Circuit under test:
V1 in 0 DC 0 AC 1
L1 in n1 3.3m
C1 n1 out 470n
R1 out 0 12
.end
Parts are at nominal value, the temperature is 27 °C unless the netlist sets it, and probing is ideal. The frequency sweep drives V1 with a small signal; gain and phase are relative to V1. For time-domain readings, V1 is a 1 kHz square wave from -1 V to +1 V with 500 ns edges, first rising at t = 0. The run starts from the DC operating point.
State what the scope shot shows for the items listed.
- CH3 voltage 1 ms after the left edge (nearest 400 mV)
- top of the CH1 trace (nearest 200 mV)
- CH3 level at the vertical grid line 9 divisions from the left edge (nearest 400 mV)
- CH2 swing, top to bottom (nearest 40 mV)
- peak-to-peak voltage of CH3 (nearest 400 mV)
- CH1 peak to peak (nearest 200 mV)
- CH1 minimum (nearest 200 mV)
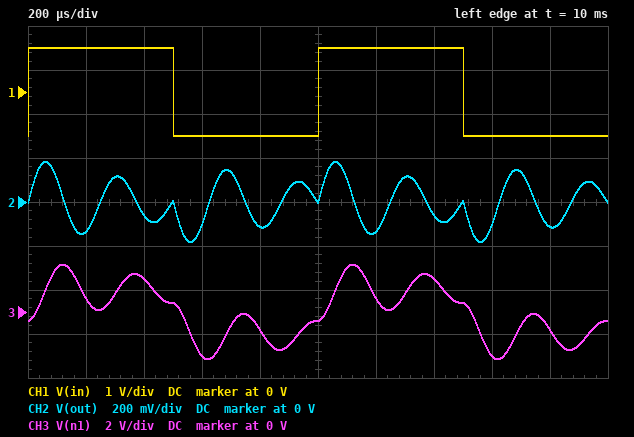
-400 mV
1.0 V
-800 mV
360 mV
4.4 V
2.0 V
-1.0 V
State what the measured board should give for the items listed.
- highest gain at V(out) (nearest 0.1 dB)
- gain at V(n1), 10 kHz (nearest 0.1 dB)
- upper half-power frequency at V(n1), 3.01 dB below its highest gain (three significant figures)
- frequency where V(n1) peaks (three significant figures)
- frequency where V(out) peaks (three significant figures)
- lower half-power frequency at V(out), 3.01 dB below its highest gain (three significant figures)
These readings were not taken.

0 dB
-13.7 dB
4.30 kHz
4.02 kHz
4.04 kHz
3.76 kHz
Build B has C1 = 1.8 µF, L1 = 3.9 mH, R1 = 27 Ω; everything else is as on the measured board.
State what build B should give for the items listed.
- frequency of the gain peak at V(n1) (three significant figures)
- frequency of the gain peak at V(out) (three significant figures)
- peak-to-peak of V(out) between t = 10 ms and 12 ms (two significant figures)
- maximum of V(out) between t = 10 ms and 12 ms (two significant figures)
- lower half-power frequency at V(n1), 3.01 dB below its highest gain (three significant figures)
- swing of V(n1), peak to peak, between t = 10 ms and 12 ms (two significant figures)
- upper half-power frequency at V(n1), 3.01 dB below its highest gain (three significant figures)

1.77 kHz
1.90 kHz
1.4 V
700 mV
1.13 kHz
3.6 V
2.30 kHz
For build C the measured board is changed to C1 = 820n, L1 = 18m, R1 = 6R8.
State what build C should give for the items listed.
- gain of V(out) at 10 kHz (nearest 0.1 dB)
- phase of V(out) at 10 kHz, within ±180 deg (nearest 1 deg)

-44.3 dB
-90 deg
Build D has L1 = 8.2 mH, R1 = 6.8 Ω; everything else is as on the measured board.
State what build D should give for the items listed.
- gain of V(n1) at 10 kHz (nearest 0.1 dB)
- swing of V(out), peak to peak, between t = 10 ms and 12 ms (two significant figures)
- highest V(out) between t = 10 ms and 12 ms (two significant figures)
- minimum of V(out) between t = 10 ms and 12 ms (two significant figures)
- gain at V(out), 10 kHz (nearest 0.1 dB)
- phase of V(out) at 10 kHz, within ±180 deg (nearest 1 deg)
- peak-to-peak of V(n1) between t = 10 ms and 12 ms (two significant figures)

-22.9 dB
170 mV
85 mV
-84 mV
-37.0 dB
-89 deg
5.1 V
